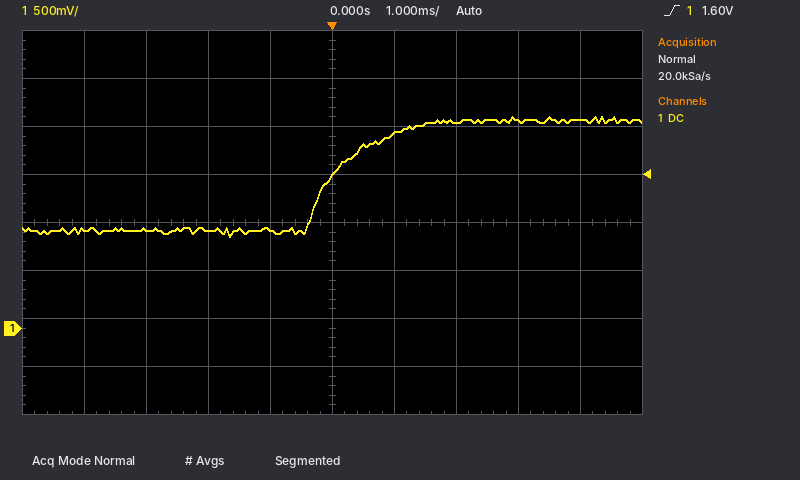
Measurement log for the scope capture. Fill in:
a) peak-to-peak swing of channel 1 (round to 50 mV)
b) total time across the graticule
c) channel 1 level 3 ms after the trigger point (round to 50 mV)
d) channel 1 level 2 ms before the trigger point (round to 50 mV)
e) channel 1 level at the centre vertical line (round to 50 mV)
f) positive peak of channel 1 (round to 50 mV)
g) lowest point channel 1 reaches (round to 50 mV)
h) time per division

1.25 V
10 ms
2.15 V
1.00 V
1.60 V
2.20 V
950 mV
1 ms
